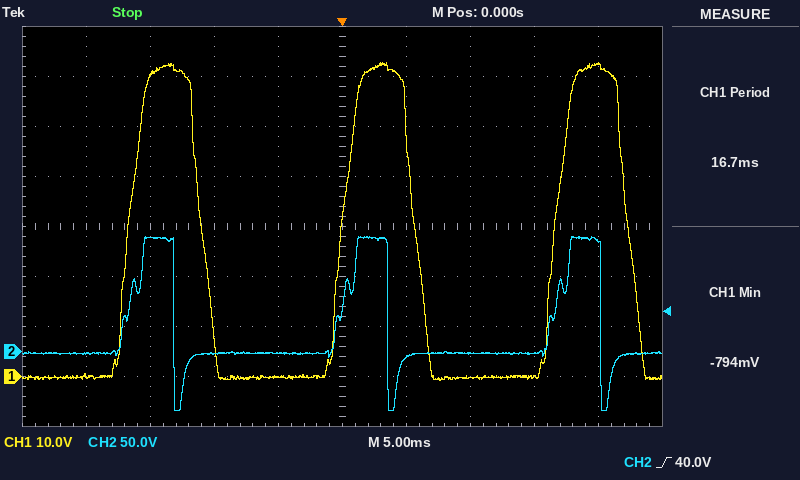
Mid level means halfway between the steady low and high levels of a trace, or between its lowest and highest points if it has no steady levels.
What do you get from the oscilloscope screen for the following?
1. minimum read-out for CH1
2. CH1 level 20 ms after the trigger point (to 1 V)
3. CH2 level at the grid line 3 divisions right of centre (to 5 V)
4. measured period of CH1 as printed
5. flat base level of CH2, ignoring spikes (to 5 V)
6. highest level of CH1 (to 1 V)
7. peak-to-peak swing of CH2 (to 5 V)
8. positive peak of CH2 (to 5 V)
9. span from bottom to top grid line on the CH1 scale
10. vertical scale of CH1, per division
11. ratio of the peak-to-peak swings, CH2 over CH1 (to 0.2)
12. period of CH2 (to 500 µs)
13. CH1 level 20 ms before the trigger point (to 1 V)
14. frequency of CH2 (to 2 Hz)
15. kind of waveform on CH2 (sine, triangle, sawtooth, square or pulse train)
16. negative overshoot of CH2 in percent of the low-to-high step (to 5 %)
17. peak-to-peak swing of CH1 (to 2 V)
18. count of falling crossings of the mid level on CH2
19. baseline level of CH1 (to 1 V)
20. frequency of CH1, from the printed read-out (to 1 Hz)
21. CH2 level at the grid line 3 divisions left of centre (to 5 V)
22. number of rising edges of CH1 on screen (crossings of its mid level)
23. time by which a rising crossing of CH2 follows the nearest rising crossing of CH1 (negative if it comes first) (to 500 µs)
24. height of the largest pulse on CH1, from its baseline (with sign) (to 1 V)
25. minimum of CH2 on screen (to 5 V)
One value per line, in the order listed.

-794 mV
62 V
0 V
16.7 ms
0 V
63 V
175 V
115 V
80 V
10 V
2.8
16.5 ms
0 V
60 Hz
pulse train
50 %
64 V
3
0 V
60 Hz
115 V
3
0.0 ms
+63 V
-60 V
